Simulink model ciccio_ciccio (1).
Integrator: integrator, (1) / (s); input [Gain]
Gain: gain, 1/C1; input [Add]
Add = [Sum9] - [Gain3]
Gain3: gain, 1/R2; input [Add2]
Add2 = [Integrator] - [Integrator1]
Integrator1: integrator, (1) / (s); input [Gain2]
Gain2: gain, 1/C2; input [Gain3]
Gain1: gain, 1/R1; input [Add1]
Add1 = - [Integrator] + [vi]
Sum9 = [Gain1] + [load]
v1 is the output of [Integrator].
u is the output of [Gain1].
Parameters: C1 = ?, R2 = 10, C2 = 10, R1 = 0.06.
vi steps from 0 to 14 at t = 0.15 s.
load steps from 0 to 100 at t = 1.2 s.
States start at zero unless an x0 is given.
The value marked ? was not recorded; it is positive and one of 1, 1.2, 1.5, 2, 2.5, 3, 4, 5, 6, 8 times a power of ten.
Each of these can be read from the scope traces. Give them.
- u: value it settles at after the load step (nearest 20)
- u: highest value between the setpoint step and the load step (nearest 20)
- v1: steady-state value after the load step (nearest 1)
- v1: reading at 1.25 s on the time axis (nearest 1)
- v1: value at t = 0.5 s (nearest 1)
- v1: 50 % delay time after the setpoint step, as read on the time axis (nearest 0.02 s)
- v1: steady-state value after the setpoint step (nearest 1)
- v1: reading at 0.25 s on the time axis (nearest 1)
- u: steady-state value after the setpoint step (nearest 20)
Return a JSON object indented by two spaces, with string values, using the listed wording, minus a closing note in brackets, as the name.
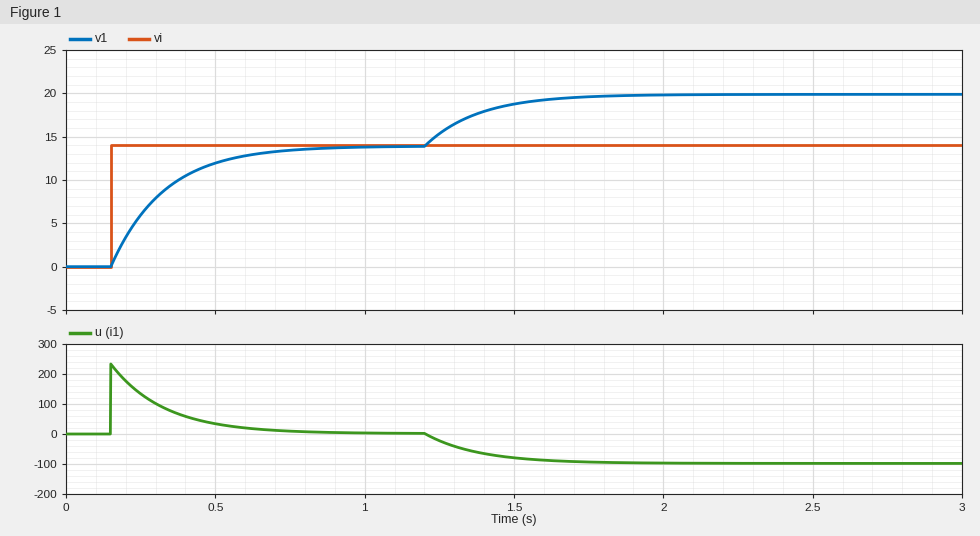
{
  "u: value it settles at after the load step": "-100",
  "u: highest value between the setpoint step and the load step": "240",
  "v1: steady-state value after the load step": "20",
  "v1: reading at 1.25 s on the time axis": "15",
  "v1: value at t = 0.5 s": "12",
  "v1: 50 % delay time after the setpoint step, as read on the time axis": "0.28 s",
  "v1: steady-state value after the setpoint step": "14",
  "v1: reading at 0.25 s on the time axis": "6",
  "u: steady-state value after the setpoint step": "0"
}
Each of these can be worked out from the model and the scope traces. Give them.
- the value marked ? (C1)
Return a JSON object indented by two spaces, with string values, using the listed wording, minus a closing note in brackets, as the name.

{
  "the value marked ?": "3"
}
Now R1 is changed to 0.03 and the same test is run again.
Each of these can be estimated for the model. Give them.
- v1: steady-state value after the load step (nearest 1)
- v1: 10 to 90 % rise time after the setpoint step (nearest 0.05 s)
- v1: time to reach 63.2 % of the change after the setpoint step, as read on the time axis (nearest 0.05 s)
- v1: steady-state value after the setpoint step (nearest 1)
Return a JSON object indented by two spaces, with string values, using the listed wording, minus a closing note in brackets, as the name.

{
  "v1: steady-state value after the load step": "17",
  "v1: 10 to 90 % rise time after the setpoint step": "0.20 s",
  "v1: time to reach 63.2 % of the change after the setpoint step, as read on the time axis": "0.25 s",
  "v1: steady-state value after the setpoint step": "14"
}
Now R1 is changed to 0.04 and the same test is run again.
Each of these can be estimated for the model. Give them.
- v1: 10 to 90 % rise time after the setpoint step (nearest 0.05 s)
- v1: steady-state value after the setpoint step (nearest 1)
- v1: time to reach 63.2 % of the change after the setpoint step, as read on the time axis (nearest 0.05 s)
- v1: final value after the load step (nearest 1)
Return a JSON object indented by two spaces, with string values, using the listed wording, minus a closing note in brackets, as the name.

{
  "v1: 10 to 90 % rise time after the setpoint step": "0.25 s",
  "v1: steady-state value after the setpoint step": "14",
  "v1: time to reach 63.2 % of the change after the setpoint step, as read on the time axis": "0.25 s",
  "v1: final value after the load step": "18"
}
